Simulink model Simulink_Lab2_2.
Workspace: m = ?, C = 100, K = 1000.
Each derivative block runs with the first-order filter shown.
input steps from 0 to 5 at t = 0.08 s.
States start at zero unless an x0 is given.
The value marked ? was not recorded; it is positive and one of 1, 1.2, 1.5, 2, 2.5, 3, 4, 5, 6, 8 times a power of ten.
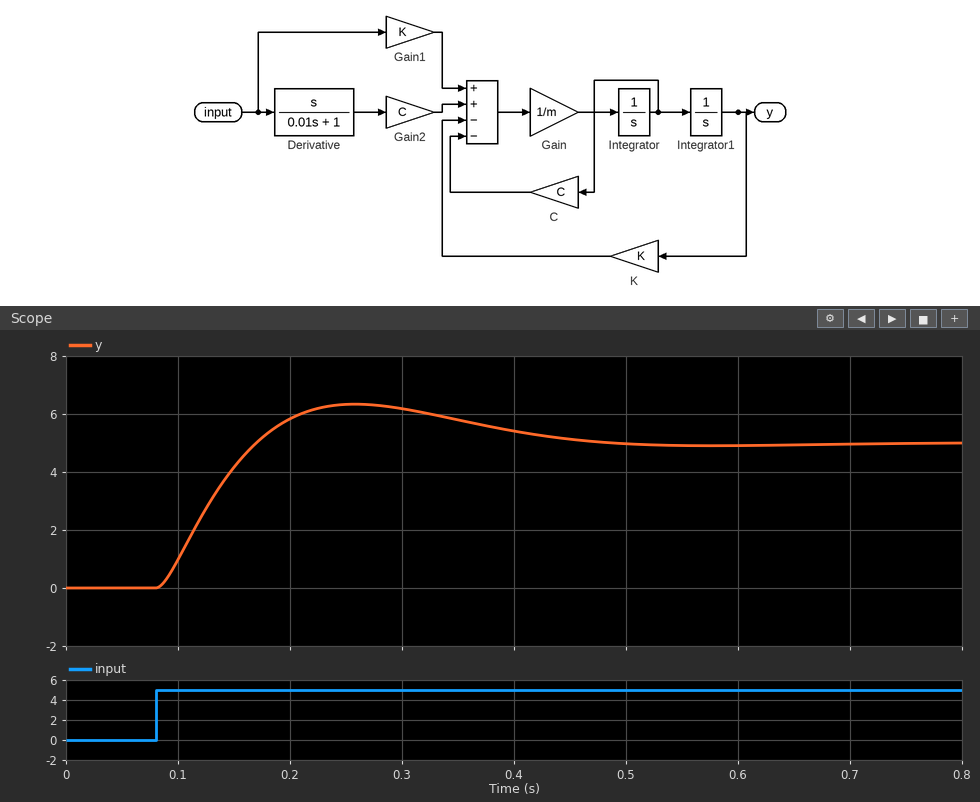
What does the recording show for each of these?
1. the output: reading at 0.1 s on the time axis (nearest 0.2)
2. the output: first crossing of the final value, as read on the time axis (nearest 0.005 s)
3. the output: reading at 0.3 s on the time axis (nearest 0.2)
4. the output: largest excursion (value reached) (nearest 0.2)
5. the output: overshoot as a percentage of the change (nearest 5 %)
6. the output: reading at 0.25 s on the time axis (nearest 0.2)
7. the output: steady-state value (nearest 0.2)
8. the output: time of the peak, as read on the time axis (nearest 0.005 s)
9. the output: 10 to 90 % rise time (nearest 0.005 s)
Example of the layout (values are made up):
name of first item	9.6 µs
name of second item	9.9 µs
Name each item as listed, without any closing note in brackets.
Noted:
the output: reading at 0.1 s on the time axis	1.0
the output: first crossing of the final value, as read on the time axis	0.170 s
the output: reading at 0.3 s on the time axis	6.2
the output: largest excursion (value reached)	6.4
the output: overshoot as a percentage of the change	25 %
the output: reading at 0.25 s on the time axis	6.4
the output: steady-state value	5.0
the output: time of the peak, as read on the time axis	0.260 s
the output: 10 to 90 % rise time	0.065 s
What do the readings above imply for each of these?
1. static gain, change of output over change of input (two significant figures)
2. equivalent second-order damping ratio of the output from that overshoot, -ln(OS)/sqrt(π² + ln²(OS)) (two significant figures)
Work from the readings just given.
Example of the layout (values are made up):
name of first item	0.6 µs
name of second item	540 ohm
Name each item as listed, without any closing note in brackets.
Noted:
static gain, change of output over change of input	1.0
equivalent second-order damping ratio of the output from that overshoot, -ln(OS)/sqrt(π² + ln²(OS))	0.40
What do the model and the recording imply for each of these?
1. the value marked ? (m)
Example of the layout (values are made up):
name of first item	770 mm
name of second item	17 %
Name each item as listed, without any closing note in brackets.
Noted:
the value marked ?	6
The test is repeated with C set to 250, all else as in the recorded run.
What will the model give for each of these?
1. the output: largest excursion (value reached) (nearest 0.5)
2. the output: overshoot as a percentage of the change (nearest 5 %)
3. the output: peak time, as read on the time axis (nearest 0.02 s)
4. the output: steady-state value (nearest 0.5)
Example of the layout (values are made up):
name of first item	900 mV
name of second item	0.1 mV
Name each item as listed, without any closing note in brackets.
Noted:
the output: largest excursion (value reached)	5.5
the output: overshoot as a percentage of the change	10 %
the output: peak time, as read on the time axis	0.22 s
the output: steady-state value	5.0
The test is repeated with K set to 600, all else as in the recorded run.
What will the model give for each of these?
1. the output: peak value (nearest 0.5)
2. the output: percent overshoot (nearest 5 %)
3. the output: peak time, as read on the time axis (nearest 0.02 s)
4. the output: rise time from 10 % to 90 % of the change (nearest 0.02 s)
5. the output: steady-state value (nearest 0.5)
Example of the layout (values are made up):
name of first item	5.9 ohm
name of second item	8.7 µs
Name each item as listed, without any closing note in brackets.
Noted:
the output: peak value	6.0
the output: percent overshoot	20 %
the output: peak time, as read on the time axis	0.30 s
the output: rise time from 10 % to 90 % of the change	0.08 s
the output: steady-state value	5.0
